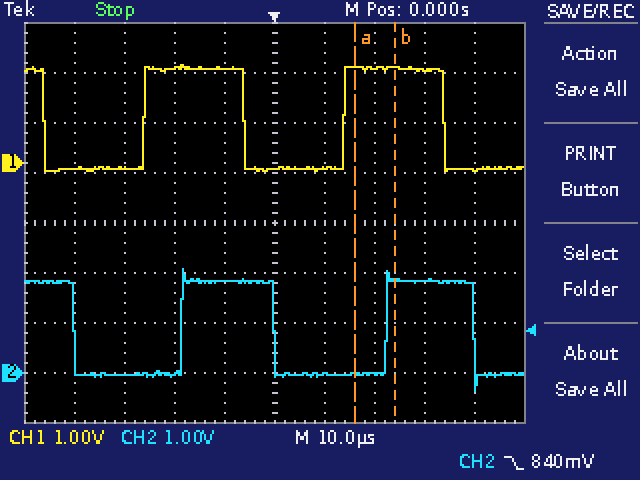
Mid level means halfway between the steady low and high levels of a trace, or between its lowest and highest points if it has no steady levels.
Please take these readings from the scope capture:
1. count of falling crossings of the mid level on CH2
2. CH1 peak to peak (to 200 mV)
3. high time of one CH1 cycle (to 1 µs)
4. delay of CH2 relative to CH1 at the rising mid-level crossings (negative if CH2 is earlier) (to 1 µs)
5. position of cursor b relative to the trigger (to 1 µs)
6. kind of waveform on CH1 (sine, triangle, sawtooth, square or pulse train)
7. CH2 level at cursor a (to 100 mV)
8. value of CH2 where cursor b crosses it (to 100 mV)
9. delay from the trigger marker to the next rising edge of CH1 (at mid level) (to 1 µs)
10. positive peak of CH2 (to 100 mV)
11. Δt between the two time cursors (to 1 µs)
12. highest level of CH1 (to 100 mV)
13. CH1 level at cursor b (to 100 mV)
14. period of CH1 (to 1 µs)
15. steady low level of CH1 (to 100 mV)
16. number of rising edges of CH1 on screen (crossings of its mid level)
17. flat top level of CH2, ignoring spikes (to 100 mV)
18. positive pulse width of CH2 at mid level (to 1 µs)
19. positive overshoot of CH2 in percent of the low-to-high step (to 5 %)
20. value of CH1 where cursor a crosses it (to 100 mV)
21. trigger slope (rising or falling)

3
2.2 V
20 µs
+8 µs
+24 µs
square
0.0 V
1.9 V
14 µs
2.1 V
8 µs
2.0 V
1.9 V
40 µs
-100 mV
2
1.8 V
18 µs
15 %
1.9 V
falling
